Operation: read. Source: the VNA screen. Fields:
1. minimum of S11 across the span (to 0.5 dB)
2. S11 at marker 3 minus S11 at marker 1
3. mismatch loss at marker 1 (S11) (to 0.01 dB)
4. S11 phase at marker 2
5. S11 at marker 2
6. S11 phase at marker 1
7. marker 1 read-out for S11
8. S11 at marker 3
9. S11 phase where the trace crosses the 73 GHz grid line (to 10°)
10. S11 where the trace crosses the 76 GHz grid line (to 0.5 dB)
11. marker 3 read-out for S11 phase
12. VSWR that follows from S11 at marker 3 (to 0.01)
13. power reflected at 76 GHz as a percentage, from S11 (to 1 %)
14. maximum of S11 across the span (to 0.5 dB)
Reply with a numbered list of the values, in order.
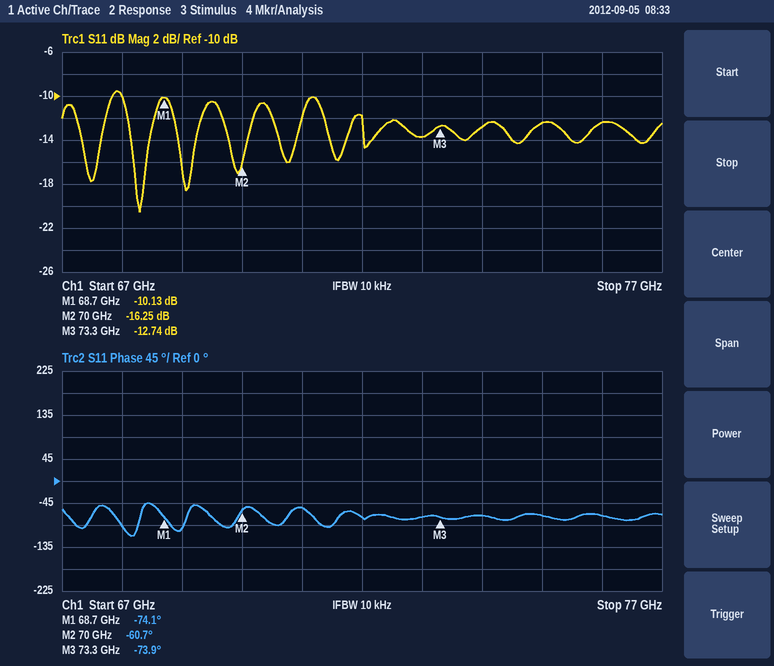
1. -20.5 dB
2. -2.61 dB
3. 0.44 dB
4. -60.7°
5. -16.25 dB
6. -74.1°
7. -10.13 dB
8. -12.74 dB
9. -70°
10. -12.5 dB
11. -73.9°
12. 1.60
13. 6 %
14. -9.5 dB
